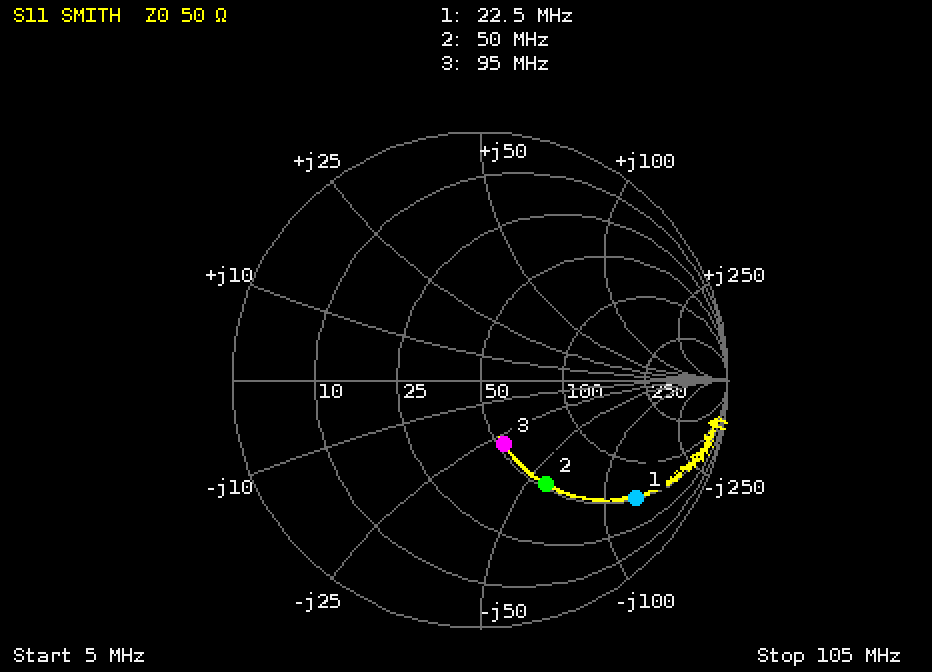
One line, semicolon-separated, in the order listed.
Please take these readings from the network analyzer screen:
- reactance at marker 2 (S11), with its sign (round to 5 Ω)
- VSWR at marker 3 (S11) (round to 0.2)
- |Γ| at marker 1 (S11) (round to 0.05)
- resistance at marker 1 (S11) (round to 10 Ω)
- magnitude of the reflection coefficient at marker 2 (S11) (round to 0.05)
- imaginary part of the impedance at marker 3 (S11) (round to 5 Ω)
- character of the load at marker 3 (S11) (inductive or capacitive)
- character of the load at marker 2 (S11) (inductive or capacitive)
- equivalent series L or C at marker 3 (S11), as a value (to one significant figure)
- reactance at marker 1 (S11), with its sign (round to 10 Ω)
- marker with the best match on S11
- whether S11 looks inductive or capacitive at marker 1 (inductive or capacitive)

-60 Ω; 1.8; 0.80; 50 Ω; 0.50; -30 Ω; capacitive; capacitive; 60 pF; -130 Ω; marker 3; capacitive
